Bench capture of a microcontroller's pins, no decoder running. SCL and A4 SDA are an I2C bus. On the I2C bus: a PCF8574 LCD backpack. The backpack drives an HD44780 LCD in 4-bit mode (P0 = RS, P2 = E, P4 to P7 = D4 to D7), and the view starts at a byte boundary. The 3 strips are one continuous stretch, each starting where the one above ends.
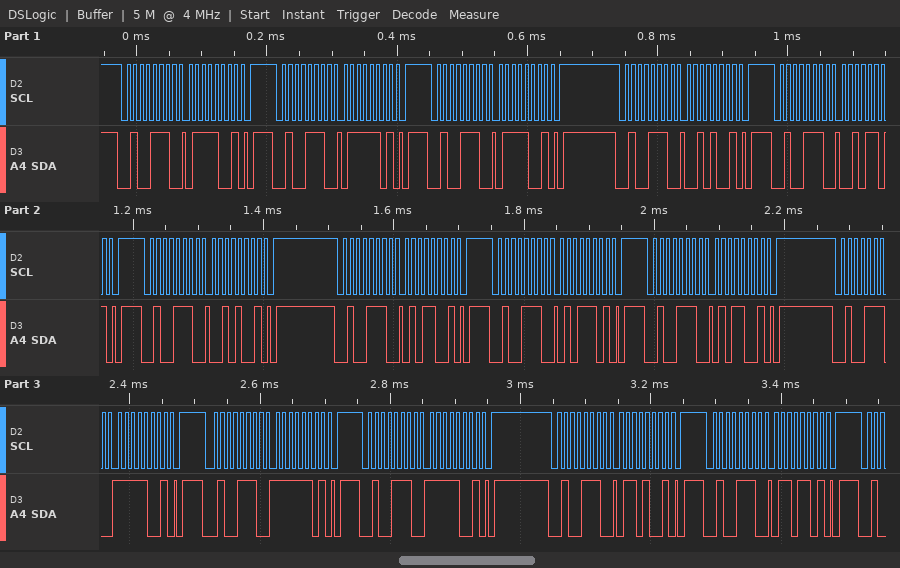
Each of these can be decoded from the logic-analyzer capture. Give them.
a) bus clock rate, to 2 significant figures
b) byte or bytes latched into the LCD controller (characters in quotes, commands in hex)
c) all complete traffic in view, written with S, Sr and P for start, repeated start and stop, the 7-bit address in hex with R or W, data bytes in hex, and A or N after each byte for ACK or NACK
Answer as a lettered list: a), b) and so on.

a) 100 kHz
b) 'r' '_'
c) S 27W A 79 A P S 27W A 7D A P S 27W A 79 A P S 27W A 29 A P S 27W A 2D A P S 27W A 29 A P S 27W A 59 A P S 27W A 5D A P S 27W A 59 A P S 27W A F9 A P S 27W A FD A P S 27W A F9 A P S 27W A 69 A P S 27W A 6D A P
